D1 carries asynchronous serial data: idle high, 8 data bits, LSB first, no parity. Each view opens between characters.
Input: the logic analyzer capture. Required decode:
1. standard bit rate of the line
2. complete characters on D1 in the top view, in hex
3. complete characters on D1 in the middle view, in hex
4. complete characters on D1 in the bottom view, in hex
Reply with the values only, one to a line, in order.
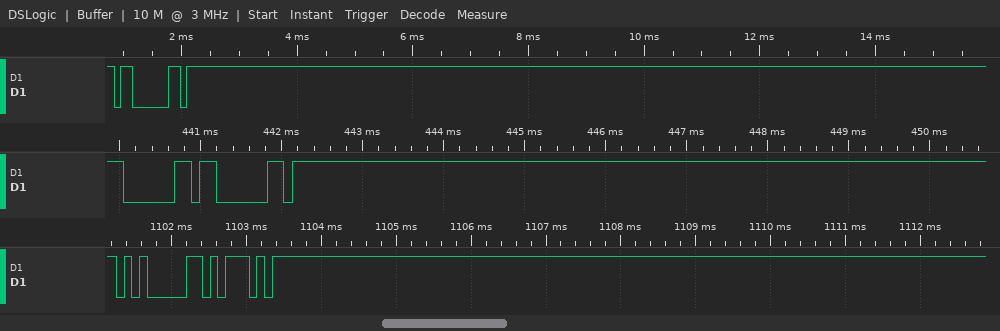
9600 baud
03, FF
60, 60
05, 5D
